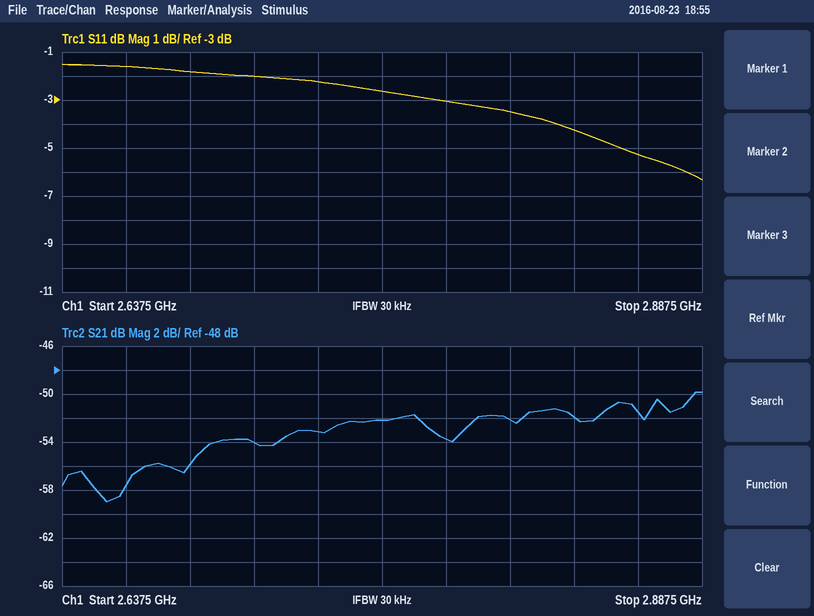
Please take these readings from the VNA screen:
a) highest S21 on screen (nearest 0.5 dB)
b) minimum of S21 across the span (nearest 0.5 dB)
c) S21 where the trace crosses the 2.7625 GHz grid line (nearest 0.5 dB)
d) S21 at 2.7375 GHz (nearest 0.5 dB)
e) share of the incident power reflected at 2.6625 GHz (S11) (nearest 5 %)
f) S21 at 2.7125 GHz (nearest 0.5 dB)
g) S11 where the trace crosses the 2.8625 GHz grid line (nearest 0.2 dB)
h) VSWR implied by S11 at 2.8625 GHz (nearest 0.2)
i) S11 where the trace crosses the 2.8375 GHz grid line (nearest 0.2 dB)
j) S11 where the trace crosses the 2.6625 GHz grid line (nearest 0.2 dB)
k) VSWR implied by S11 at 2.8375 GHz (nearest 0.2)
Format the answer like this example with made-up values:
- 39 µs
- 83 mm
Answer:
- -50.0 dB
- -59.0 dB
- -52.0 dB
- -53.0 dB
- 70 %
- -54.0 dB
- -5.2 dB
- 3.4
- -4.2 dB
- -1.6 dB
- 4.2
